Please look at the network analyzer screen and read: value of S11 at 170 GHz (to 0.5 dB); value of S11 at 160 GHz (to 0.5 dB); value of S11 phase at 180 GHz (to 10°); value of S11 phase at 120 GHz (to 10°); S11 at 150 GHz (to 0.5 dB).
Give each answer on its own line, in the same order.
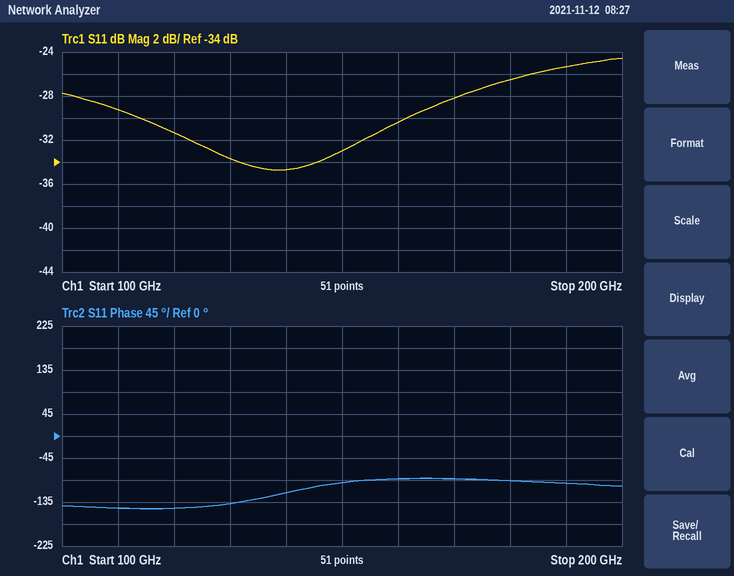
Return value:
-28.0 dB
-30.5 dB
-90°
-150°
-33.0 dB
